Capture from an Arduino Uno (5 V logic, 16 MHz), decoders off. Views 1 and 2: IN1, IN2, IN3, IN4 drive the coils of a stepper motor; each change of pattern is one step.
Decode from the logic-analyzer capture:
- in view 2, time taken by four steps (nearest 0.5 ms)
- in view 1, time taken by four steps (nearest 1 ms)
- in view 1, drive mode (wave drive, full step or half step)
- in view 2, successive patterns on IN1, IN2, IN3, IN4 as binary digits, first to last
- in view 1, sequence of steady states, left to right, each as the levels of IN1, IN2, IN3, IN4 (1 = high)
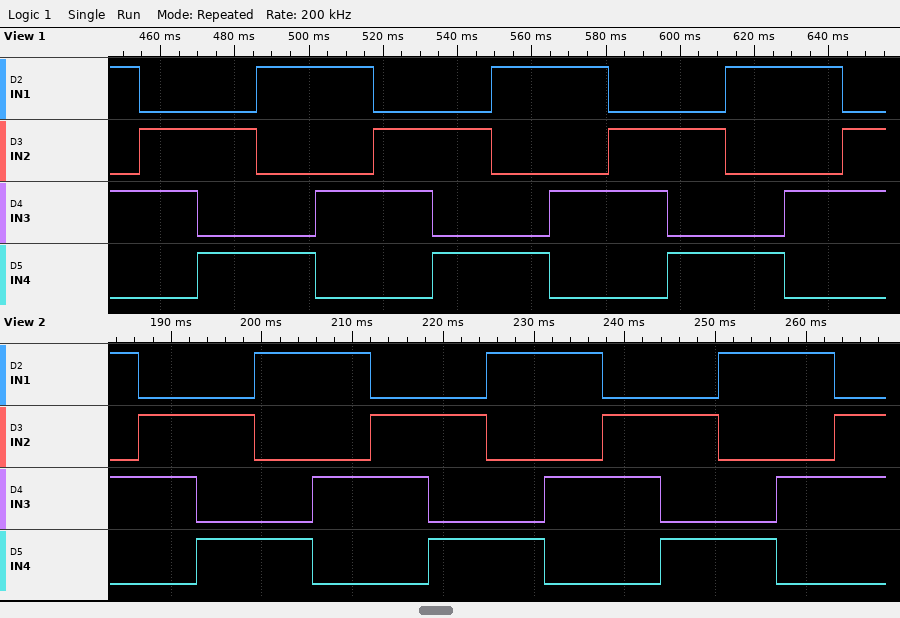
25.5 ms
63 ms
full step
1010 0110 0101 1001 1010 0110 0101 1001 1010 0110 0101 1001 1010 0110
1010 0110 0101 1001 1010 0110 0101 1001 1010 0110 0101 1001 1010 0110
